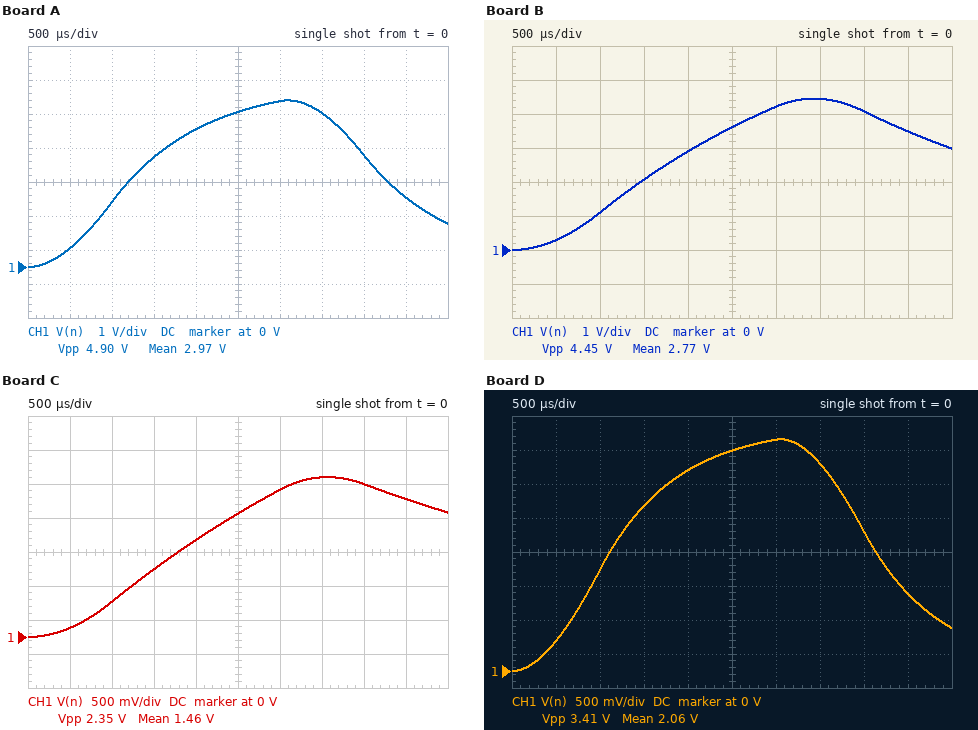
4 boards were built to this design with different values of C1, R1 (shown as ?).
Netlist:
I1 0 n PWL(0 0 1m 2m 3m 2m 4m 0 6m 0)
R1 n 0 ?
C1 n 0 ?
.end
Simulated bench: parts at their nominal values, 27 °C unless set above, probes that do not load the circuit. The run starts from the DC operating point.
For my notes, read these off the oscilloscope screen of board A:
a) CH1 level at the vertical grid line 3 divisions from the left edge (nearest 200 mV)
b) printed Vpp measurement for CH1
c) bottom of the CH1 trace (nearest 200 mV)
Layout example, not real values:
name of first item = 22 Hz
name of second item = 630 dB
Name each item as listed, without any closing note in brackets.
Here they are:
CH1 level at the vertical grid line 3 divisions from the left edge = 3.2 V
printed Vpp measurement for CH1 = 4.90 V
bottom of the CH1 trace = 0 V
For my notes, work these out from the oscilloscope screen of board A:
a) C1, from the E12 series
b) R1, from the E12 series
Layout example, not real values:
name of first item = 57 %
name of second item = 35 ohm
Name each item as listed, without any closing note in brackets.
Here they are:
C1, from the E12 series = 390 nF
R1, from the E12 series = 2.7 kΩ
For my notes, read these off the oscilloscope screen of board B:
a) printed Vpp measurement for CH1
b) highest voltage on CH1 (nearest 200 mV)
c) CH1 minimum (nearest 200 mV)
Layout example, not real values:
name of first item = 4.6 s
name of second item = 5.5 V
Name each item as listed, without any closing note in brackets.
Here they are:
printed Vpp measurement for CH1 = 4.45 V
highest voltage on CH1 = 4.4 V
CH1 minimum = 0 V
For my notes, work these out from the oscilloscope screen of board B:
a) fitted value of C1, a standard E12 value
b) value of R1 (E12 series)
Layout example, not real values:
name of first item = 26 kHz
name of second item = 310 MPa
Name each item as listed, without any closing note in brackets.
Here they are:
fitted value of C1, a standard E12 value = 820 nF
value of R1 = 3.9 kΩ
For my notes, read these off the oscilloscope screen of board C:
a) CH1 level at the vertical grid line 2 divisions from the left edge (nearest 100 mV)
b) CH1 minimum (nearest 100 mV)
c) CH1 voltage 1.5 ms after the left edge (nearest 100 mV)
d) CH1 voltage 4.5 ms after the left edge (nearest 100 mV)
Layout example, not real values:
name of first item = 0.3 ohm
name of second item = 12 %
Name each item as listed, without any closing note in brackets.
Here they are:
CH1 level at the vertical grid line 2 divisions from the left edge = 500 mV
CH1 minimum = 0 V
CH1 voltage 1.5 ms after the left edge = 1.0 V
CH1 voltage 4.5 ms after the left edge = 2.0 V
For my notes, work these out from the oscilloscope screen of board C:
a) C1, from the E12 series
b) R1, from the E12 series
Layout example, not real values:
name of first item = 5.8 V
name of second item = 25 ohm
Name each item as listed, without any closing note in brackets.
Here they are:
C1, from the E12 series = 1.8 µF
R1, from the E12 series = 2.7 kΩ
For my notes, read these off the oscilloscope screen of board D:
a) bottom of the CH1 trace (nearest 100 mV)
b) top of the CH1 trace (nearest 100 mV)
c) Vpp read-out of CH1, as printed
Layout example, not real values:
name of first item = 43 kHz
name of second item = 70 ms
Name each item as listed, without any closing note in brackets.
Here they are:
bottom of the CH1 trace = 0 V
top of the CH1 trace = 3.4 V
Vpp read-out of CH1, as printed = 3.41 V
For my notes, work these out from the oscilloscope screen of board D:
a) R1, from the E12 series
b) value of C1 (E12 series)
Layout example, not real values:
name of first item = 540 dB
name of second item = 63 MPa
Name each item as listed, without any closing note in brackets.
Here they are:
R1, from the E12 series = 1.8 kΩ
value of C1 = 470 nF
